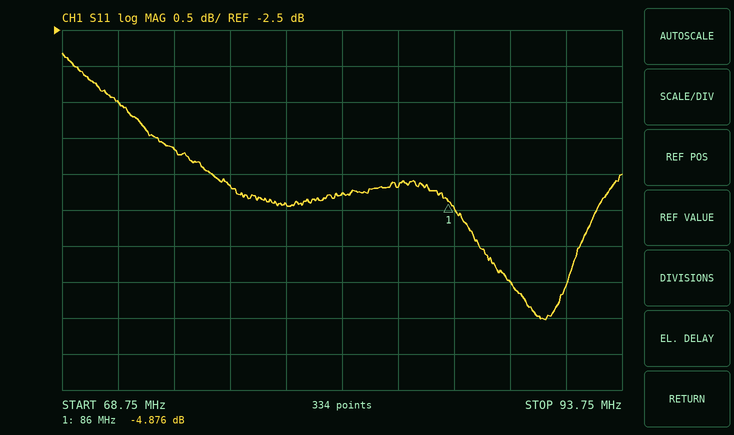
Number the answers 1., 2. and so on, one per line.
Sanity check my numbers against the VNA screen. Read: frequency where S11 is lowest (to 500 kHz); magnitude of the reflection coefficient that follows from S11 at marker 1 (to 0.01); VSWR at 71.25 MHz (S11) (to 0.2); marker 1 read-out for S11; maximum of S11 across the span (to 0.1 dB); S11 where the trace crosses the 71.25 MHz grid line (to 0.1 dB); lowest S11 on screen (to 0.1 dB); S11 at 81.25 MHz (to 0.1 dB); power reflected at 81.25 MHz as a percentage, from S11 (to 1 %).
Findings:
1. 90.5 MHz
2. 0.57
3. 5.0
4. -4.876 dB
5. -2.8 dB
6. -3.5 dB
7. -6.5 dB
8. -4.8 dB
9. 33 %
